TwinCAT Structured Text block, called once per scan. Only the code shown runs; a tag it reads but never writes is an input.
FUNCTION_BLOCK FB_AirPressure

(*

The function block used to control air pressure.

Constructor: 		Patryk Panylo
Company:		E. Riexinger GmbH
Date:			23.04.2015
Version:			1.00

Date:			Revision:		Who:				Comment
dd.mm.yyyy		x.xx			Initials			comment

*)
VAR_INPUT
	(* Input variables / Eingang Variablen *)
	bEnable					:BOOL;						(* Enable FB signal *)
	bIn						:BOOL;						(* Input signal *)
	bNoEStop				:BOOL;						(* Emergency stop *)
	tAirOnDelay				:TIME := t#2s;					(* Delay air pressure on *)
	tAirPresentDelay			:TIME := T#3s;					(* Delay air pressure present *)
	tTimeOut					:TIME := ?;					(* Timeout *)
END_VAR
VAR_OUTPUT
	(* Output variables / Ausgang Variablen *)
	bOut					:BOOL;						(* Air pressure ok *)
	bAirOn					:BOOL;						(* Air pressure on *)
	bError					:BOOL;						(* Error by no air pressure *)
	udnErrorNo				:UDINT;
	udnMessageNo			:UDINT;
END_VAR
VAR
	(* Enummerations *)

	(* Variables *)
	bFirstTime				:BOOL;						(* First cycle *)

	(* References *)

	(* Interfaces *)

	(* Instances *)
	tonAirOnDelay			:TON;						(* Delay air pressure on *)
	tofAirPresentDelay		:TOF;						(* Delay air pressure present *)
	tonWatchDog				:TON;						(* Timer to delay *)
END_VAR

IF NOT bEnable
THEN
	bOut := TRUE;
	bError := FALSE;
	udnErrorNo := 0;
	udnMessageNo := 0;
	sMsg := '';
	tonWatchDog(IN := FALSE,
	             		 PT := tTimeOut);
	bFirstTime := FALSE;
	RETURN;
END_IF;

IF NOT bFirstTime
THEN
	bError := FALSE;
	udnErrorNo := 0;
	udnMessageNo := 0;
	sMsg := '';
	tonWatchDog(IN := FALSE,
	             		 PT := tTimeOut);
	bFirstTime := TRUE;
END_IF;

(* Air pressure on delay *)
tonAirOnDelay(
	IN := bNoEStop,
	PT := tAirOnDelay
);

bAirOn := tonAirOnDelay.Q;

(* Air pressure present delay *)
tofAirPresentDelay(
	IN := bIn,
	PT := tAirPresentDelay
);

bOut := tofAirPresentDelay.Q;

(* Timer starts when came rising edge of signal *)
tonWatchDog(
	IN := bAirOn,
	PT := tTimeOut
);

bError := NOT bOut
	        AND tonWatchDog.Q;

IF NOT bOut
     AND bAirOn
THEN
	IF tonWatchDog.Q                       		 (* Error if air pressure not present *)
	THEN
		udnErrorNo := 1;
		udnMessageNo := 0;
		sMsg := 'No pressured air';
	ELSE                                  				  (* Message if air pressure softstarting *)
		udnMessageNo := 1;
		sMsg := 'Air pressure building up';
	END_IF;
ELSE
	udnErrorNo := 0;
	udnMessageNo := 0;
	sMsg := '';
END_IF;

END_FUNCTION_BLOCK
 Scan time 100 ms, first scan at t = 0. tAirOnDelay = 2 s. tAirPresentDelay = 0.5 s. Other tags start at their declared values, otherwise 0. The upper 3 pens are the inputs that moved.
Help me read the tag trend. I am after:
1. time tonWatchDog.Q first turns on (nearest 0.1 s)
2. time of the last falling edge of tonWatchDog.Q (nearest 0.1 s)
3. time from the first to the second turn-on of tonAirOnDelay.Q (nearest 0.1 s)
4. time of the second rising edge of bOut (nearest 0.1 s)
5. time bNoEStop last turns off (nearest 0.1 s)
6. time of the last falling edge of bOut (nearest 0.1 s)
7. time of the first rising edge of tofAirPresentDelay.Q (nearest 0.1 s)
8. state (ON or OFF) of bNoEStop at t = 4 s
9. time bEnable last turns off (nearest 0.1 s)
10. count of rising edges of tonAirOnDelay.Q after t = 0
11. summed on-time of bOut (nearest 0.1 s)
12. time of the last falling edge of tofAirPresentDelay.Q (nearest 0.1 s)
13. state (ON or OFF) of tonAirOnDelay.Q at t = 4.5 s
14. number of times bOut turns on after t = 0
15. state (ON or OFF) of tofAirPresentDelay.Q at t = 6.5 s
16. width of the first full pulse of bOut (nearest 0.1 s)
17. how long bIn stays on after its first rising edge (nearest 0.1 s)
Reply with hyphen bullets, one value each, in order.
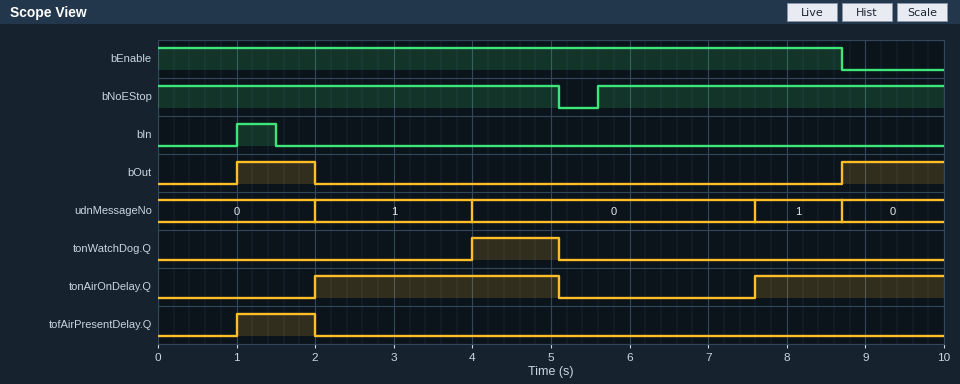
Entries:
- 4.0 s
- 5.1 s
- 5.6 s
- 8.7 s
- 5.1 s
- 2.0 s
- 1.0 s
- ON
- 8.7 s
- 2
- 2.3 s
- 2.0 s
- ON
- 2
- OFF
- 1.0 s
- 0.5 s
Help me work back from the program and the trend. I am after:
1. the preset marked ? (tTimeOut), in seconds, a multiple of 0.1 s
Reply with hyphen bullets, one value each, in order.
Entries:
- 2.0 s
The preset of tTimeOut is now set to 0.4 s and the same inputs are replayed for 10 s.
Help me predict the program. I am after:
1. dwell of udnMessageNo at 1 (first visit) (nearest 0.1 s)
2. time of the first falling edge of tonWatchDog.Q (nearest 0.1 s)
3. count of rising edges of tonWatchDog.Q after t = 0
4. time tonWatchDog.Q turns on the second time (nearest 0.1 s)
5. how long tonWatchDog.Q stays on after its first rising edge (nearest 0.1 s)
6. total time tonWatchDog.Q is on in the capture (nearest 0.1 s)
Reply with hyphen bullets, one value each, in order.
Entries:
- 0.4 s
- 5.1 s
- 2
- 8.0 s
- 2.7 s
- 3.4 s
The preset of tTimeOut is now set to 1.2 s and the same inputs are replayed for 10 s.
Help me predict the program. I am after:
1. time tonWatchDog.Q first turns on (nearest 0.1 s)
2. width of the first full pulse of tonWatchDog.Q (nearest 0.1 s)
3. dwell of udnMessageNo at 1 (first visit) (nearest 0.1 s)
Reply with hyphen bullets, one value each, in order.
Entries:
- 3.2 s
- 1.9 s
- 1.2 s
